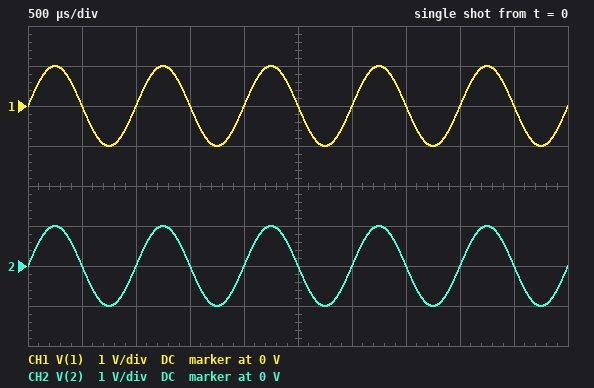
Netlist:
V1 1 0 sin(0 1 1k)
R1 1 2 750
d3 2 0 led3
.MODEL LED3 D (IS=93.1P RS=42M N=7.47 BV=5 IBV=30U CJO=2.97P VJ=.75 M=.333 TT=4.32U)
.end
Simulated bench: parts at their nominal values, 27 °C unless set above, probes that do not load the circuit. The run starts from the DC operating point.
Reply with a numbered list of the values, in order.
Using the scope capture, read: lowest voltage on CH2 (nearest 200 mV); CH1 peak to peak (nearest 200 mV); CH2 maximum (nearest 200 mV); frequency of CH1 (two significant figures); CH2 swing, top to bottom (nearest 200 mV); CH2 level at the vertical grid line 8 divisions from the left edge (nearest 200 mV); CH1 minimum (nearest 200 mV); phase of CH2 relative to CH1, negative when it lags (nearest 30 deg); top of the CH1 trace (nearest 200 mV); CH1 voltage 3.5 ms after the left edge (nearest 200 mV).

1. -1.0 V
2. 2.0 V
3. 1.0 V
4. 1.0 kHz
5. 2.0 V
6. 0 V
7. -1.0 V
8. 0 deg
9. 1.0 V
10. 0 V
